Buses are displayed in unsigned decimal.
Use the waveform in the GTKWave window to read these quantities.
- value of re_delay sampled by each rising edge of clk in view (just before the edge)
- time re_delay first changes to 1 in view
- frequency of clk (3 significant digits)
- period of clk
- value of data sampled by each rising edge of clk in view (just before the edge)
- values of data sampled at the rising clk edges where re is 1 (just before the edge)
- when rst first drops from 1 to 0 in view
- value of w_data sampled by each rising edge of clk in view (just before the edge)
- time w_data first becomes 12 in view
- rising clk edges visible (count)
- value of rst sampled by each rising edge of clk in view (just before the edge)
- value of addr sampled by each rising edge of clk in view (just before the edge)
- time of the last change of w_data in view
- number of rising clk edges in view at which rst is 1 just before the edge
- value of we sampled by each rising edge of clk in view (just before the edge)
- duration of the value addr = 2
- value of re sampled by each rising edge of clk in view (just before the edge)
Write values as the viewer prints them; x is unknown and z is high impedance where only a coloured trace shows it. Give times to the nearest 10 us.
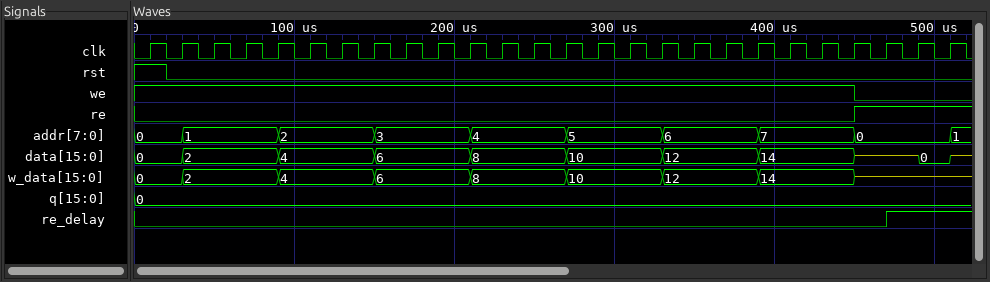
0 0 0 0 0 0 0 0 0 0 0 0 0 0 0 0 0 0 0 0 0 0 0 0 1 1
470 us
50.0 kHz
20 us
0, 0, 2, 2, 2, 4, 4, 4, 6, 6, 6, 8, 8, 8, 10, 10, 10, 12, 12, 12, 14, 14, 14, z, z, 0
z, z, 0
20 us
0, 0, 2, 2, 2, 4, 4, 4, 6, 6, 6, 8, 8, 8, 10, 10, 10, 12, 12, 12, 14, 14, 14, z, z, z
330 us
26
1 0 0 0 0 0 0 0 0 0 0 0 0 0 0 0 0 0 0 0 0 0 0 0 0 0
0, 0, 1, 1, 1, 2, 2, 2, 3, 3, 3, 4, 4, 4, 5, 5, 5, 6, 6, 6, 7, 7, 7, 0, 0, 0
450 us
1
1 1 1 1 1 1 1 1 1 1 1 1 1 1 1 1 1 1 1 1 1 1 1 0 0 0
60 us
0 0 0 0 0 0 0 0 0 0 0 0 0 0 0 0 0 0 0 0 0 0 0 1 1 1
